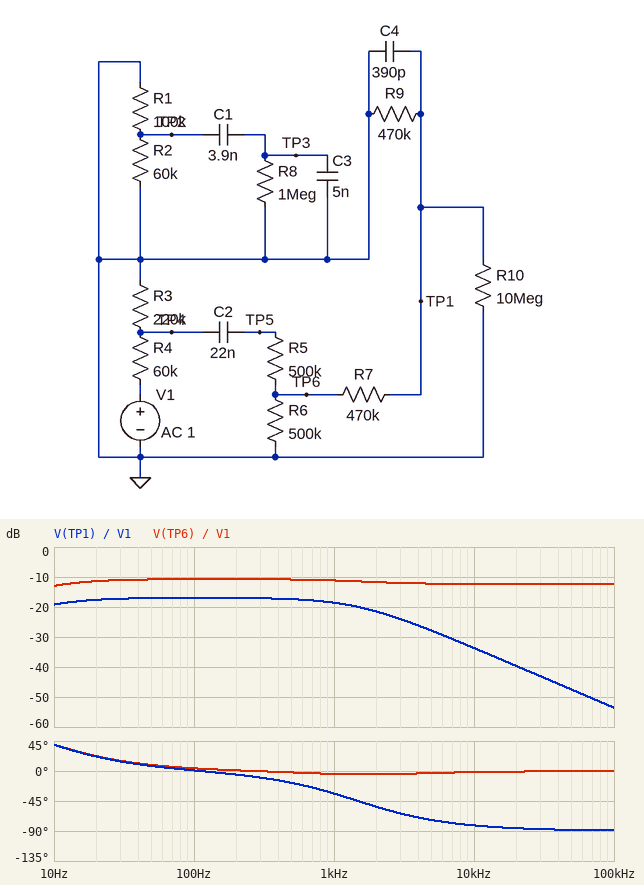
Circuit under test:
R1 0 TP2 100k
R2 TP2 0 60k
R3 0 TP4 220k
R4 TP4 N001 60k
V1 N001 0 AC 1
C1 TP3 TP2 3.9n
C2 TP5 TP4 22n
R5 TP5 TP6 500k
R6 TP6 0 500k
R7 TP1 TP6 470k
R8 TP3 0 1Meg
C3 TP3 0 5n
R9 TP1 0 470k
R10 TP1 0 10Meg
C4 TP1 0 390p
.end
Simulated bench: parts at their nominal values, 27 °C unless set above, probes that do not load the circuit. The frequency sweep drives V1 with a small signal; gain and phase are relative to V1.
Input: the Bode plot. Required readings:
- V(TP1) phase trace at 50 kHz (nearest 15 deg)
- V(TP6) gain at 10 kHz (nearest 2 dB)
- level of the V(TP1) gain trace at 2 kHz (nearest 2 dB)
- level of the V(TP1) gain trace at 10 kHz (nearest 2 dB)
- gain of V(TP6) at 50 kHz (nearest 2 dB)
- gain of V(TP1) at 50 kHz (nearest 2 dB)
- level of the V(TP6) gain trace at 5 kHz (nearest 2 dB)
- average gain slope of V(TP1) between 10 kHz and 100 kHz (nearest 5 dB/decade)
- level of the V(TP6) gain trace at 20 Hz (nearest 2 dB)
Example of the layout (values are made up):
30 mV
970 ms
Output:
-90 deg
-12 dB
-22 dB
-34 dB
-12 dB
-48 dB
-12 dB
-20 dB/decade
-12 dB
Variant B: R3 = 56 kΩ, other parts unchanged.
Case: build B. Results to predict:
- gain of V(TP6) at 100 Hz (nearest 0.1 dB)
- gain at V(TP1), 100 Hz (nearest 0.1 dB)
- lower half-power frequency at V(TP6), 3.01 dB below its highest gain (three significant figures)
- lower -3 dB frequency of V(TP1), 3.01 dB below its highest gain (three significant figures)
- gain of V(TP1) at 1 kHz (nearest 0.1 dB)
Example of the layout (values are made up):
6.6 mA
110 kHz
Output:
-14.8 dB
-21.0 dB
8.42 Hz
8.38 Hz
-22.6 dB
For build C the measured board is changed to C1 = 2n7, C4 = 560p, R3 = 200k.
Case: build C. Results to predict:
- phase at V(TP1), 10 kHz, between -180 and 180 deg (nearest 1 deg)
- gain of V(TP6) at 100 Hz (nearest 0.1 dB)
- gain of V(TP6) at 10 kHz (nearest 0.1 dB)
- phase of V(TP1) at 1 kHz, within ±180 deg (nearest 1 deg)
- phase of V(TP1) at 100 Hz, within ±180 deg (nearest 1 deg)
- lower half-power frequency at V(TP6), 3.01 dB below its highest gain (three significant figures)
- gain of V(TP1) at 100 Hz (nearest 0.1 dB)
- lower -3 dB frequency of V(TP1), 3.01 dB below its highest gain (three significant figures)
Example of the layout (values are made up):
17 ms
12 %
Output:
-84 deg
-10.9 dB
-12.5 dB
-44 deg
-1 deg
8.23 Hz
-17.2 dB
8.18 Hz
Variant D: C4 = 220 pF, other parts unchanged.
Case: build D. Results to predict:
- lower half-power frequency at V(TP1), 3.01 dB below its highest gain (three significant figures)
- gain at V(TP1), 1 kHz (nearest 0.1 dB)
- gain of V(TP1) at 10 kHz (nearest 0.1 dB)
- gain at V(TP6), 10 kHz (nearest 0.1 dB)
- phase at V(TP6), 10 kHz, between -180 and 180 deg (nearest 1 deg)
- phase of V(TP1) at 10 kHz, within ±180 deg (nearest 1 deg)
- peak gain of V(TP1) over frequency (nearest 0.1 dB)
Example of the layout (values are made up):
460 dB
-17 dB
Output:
8.25 Hz
-17.5 dB
-28.9 dB
-12.2 dB
-3 deg
-75 deg
-16.9 dB
